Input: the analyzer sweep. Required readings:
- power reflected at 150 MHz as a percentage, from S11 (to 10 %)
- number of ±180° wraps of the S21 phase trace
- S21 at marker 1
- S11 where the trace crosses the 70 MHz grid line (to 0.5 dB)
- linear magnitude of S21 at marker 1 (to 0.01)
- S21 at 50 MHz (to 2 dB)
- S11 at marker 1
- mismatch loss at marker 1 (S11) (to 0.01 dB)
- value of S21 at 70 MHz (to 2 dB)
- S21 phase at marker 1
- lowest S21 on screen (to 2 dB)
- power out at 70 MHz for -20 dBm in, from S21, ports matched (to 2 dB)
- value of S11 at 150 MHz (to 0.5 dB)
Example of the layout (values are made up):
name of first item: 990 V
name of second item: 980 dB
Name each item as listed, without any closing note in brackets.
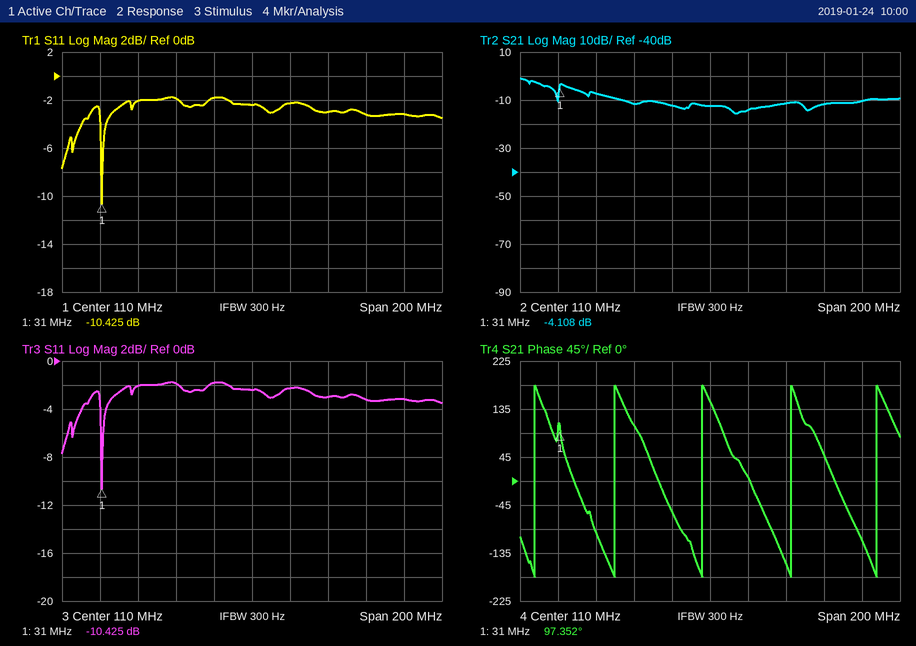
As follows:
power reflected at 150 MHz as a percentage, from S11: 50 %
number of ±180° wraps of the S21 phase trace: 5
S21 at marker 1: -4.108 dB
S11 where the trace crosses the 70 MHz grid line: -2.0 dB
linear magnitude of S21 at marker 1: 0.62
S21 at 50 MHz: -8 dB
S11 at marker 1: -10.425 dB
mismatch loss at marker 1 (S11): 0.41 dB
value of S21 at 70 MHz: -12 dB
S21 phase at marker 1: 97.352°
lowest S21 on screen: -16 dB
power out at 70 MHz for -20 dBm in, from S21, ports matched: -32 dBm
value of S11 at 150 MHz: -3.0 dB
